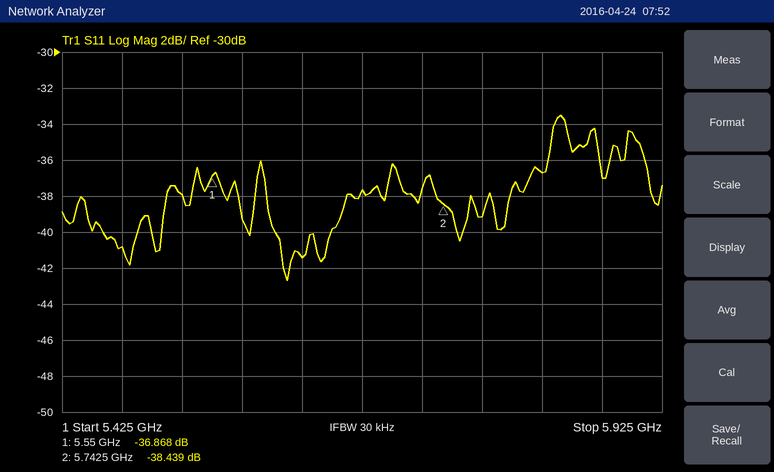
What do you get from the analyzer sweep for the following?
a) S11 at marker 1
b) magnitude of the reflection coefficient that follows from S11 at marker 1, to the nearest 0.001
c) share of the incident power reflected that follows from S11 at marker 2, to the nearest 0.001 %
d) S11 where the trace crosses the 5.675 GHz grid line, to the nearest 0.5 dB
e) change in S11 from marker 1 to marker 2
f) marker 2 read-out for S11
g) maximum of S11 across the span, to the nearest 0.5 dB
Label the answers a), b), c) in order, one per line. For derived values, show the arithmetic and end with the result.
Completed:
a) -36.868 dB
b) 10^(-36.868/20) ≈ 0.014
c) 10^(-38.439/10) ≈ 0.014 %
d) -37.5 dB
e) -38.439 − (-36.868) = -1.571 dB
f) -38.439 dB
g) -33.5 dB
